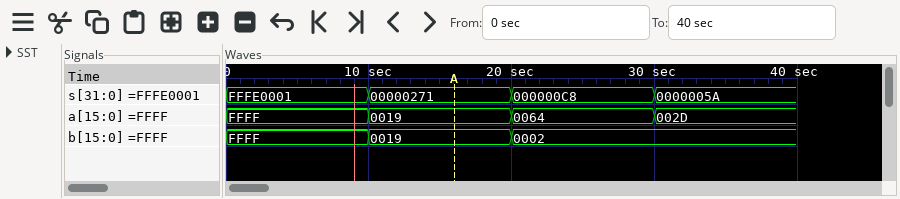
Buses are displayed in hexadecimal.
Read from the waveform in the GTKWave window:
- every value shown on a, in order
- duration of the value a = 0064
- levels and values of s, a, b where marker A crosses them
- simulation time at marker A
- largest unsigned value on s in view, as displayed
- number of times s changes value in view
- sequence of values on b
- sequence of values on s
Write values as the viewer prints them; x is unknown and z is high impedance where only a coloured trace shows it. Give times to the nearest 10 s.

FFFF, 0019, 0064, 002D
10 s
s=00000271, a=0019, b=0019
20 s
FFFE0001
3
FFFF, 0019, 0002
FFFE0001, 00000271, 000000C8, 0000005A
